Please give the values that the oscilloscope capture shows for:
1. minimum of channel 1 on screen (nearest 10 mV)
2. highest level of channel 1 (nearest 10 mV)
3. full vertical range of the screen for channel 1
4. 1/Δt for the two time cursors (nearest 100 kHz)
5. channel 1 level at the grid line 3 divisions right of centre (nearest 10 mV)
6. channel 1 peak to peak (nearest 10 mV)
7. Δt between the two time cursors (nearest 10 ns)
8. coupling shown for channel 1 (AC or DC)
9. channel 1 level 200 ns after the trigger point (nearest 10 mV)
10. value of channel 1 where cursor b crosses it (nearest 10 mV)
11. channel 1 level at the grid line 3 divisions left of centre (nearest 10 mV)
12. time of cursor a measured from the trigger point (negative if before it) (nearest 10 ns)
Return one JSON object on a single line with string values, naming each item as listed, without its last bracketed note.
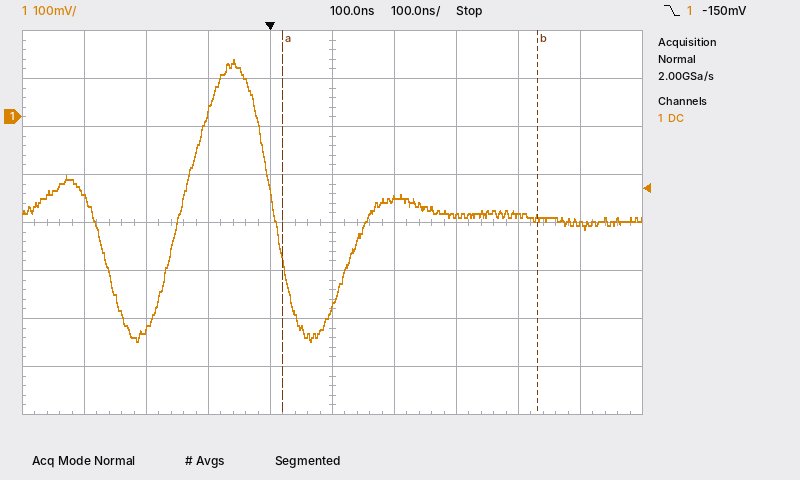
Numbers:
{"minimum of channel 1 on screen": "-470 mV", "highest level of channel 1": "120 mV", "full vertical range of the screen for channel 1": "800 mV", "1/Δt for the two time cursors": "2.4 MHz", "channel 1 level at the grid line 3 divisions right of centre": "-210 mV", "channel 1 peak to peak": "590 mV", "Δt between the two time cursors": "410 ns", "coupling shown for channel 1": "DC", "channel 1 level 200 ns after the trigger point": "-170 mV", "value of channel 1 where cursor b crosses it": "-210 mV", "channel 1 level at the grid line 3 divisions left of centre": "-440 mV", "time of cursor a measured from the trigger point (negative if before it)": "+20 ns"}
